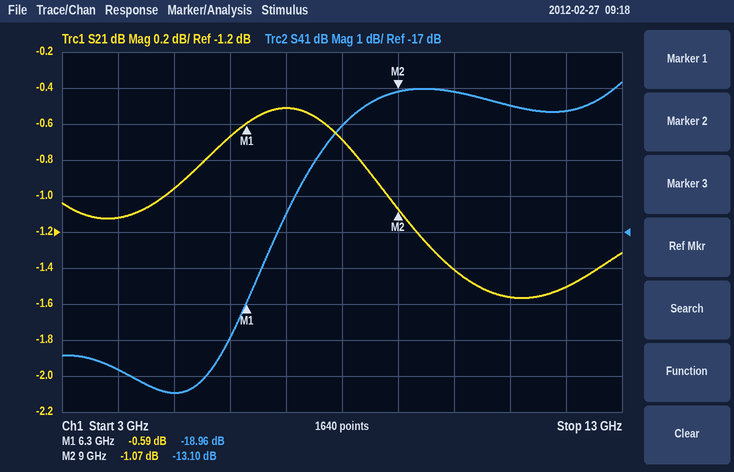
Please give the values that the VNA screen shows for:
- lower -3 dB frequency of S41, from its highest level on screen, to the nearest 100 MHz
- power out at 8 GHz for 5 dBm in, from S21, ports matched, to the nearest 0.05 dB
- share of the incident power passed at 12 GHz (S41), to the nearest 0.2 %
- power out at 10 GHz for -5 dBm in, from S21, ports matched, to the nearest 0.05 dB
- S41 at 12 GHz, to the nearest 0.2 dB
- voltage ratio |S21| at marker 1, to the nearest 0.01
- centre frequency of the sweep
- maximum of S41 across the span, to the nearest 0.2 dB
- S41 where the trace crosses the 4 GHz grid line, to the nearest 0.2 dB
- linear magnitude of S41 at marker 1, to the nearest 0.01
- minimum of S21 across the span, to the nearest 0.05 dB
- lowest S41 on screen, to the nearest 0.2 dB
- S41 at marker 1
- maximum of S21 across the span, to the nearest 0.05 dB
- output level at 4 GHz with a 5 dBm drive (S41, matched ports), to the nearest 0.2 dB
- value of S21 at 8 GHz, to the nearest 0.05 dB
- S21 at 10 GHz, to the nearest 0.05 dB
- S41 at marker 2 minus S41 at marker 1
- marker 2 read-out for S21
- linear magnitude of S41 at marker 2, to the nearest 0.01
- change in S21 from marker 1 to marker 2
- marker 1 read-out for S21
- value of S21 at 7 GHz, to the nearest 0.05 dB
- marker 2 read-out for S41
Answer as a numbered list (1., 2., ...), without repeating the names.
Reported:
1. 7.2 GHz
2. 4.30 dBm
3. 4.4 %
4. -6.40 dBm
5. -13.6 dB
6. 0.93
7. 8 GHz
8. -12.8 dB
9. -20.8 dB
10. 0.11
11. -1.55 dB
12. -21.4 dB
13. -18.96 dB
14. -0.50 dB
15. -15.8 dBm
16. -0.70 dB
17. -1.40 dB
18. 5.86 dB
19. -1.07 dB
20. 0.22
21. -0.48 dB
22. -0.59 dB
23. -0.50 dB
24. -13.10 dB
